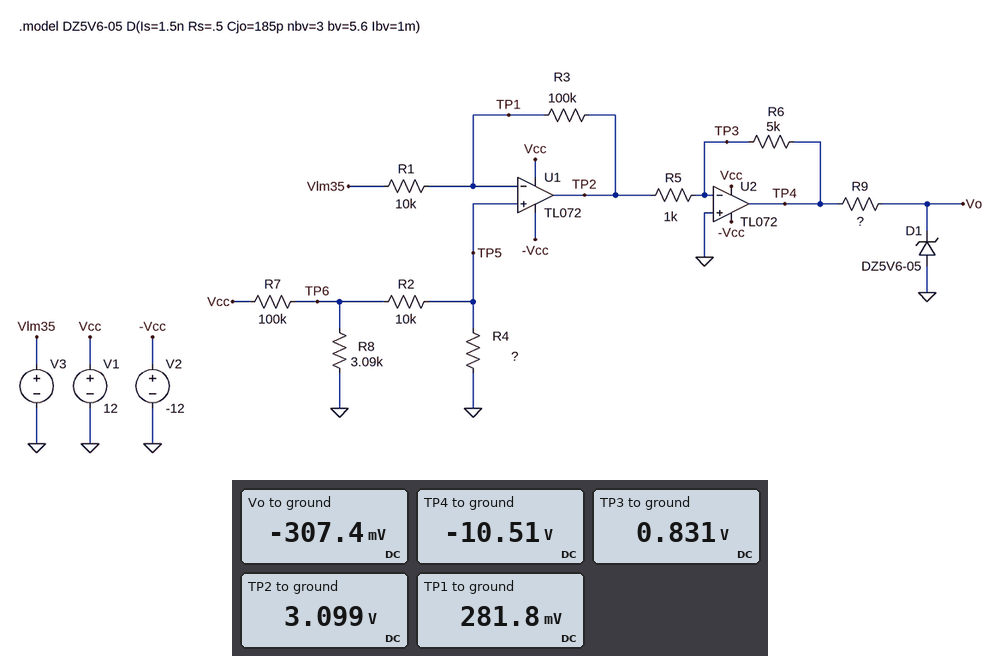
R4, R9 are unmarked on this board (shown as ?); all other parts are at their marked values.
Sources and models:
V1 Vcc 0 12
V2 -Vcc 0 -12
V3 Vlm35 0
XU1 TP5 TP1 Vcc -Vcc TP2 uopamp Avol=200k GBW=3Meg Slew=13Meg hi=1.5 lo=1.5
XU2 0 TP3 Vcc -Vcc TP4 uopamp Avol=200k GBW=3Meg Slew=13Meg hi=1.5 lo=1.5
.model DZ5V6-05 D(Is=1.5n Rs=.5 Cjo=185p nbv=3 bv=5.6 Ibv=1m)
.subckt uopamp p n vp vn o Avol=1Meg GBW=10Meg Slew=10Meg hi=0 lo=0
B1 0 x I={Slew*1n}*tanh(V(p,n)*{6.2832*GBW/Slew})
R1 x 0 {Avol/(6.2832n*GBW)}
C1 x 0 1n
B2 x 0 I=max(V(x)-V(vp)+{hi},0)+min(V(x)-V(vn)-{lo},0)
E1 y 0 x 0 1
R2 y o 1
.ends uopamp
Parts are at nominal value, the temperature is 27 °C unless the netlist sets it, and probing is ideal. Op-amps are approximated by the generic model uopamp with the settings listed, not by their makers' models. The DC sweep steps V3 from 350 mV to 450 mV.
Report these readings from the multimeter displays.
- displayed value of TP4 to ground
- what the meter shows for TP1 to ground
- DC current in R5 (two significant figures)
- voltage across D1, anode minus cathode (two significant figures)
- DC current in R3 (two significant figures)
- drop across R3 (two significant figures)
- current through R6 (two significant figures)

-10.51 V
281.8 mV
2.3 mA
310 mV
28 µA
2.8 V
2.3 mA
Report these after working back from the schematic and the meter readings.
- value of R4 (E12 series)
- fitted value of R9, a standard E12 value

47 kΩ
47 kΩ
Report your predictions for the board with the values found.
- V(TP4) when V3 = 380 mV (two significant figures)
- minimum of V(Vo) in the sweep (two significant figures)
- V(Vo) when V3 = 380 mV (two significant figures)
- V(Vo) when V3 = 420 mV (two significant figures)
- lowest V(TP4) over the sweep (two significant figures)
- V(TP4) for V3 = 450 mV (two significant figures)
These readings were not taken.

3.5 V
2.0 V
3.5 V
5.2 V
2.0 V
7.0 V
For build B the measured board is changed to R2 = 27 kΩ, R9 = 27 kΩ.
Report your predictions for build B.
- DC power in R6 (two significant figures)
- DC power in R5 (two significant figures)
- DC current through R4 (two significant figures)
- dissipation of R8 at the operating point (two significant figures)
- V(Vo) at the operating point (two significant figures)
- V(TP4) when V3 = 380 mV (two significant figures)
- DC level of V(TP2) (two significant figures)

23 mW
4.6 mW
4.7 µA
39 µW
-320 mV
6.9 V
2.4 V
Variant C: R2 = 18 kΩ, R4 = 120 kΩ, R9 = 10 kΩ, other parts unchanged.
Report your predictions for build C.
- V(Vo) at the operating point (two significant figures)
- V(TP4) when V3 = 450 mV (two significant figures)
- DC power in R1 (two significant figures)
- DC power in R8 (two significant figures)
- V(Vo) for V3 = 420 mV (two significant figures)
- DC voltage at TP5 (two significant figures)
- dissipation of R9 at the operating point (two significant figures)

-350 mV
5.7 V
9.4 µW
40 µW
4.2 V
310 mV
10 mW
